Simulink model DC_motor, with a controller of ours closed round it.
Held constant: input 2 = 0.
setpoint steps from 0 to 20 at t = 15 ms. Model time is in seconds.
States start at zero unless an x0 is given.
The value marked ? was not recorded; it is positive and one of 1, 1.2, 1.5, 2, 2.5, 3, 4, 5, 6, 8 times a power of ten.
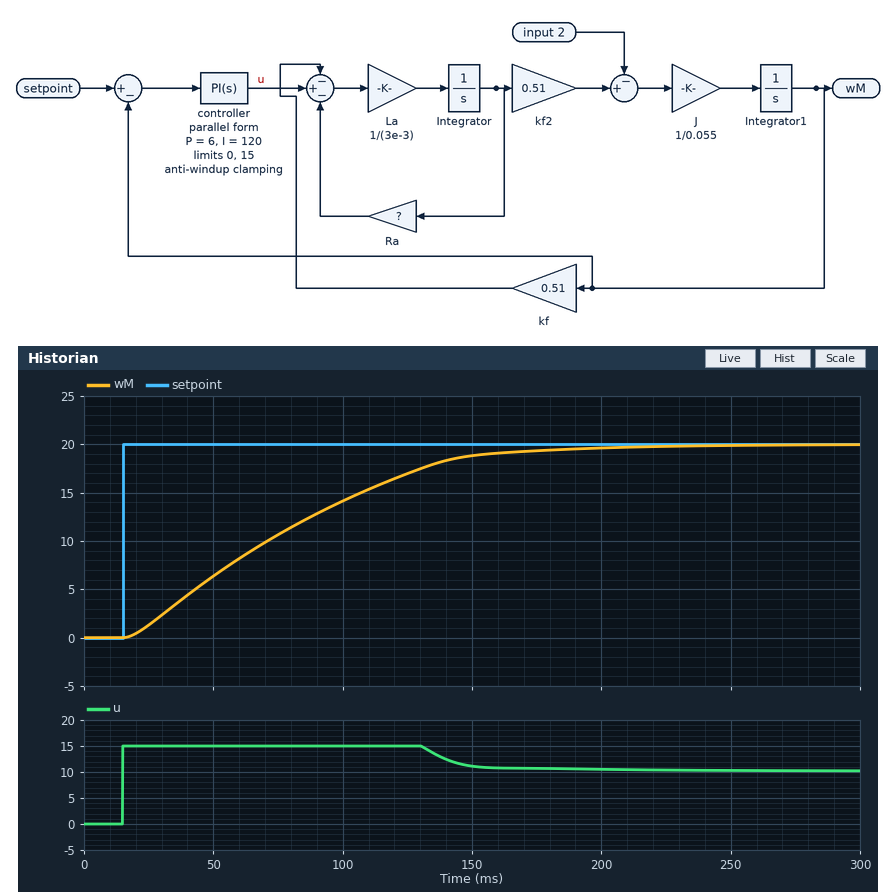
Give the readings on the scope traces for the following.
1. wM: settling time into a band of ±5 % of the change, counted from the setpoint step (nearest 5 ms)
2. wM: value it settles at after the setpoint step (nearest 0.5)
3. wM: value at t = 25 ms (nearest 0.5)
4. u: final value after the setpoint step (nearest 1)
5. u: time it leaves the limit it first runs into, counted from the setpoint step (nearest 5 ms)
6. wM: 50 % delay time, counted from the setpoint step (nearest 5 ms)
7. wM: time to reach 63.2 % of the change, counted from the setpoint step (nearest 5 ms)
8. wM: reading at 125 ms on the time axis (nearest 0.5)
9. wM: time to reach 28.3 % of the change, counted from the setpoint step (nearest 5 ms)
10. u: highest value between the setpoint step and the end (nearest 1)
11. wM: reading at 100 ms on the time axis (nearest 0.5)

140 ms
20.0
1.5
10
115 ms
55 ms
75 ms
17.0
30 ms
15
14.0
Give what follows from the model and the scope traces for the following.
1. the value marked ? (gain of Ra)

0.6
